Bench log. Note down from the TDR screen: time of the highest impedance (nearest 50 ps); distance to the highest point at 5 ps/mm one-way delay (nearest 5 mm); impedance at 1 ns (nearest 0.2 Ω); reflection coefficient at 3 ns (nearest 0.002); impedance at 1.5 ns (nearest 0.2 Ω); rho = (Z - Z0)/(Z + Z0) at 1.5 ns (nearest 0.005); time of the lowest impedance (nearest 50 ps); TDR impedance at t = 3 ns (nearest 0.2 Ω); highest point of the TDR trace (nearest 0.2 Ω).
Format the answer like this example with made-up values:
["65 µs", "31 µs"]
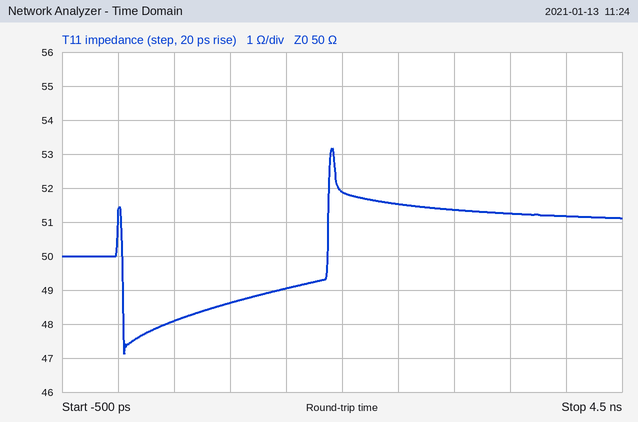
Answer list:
["1.90 ns", "190 mm", "48.6 Ω", "+0.014", "49.0 Ω", "-0.010", "50 ps", "51.4 Ω", "53.2 Ω"]
